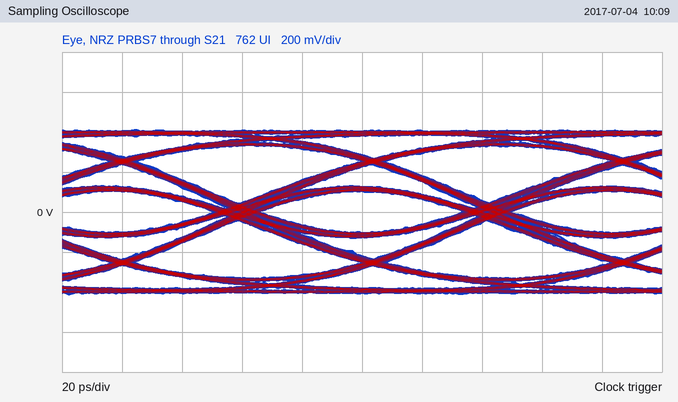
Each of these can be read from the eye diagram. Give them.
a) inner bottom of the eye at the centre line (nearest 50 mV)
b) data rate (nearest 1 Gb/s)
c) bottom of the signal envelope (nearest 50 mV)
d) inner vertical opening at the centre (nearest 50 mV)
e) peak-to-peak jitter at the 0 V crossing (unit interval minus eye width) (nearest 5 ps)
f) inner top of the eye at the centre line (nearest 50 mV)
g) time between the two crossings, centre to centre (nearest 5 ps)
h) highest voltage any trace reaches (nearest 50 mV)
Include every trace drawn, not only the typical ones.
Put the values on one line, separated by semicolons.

-100 mV; 12 Gb/s; -400 mV; 200 mV; 15 ps; 100 mV; 85 ps; 400 mV
